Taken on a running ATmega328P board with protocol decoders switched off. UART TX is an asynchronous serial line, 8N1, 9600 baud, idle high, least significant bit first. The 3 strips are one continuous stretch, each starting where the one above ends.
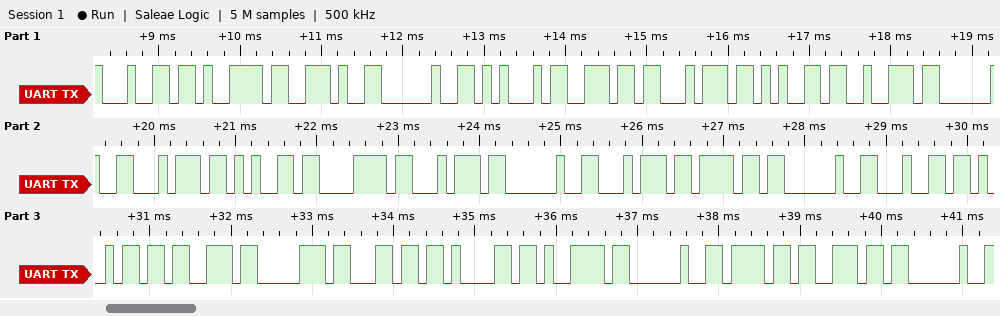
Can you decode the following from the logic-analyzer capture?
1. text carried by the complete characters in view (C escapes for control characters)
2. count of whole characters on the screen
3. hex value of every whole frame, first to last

"dy. Enter text to display on "
29
64 79 2E 20 45 6E 74 65 72 20 74 65 78 74 20 74 6F 20 64 69 73 70 6C 61 79 20 6F 6E 20
